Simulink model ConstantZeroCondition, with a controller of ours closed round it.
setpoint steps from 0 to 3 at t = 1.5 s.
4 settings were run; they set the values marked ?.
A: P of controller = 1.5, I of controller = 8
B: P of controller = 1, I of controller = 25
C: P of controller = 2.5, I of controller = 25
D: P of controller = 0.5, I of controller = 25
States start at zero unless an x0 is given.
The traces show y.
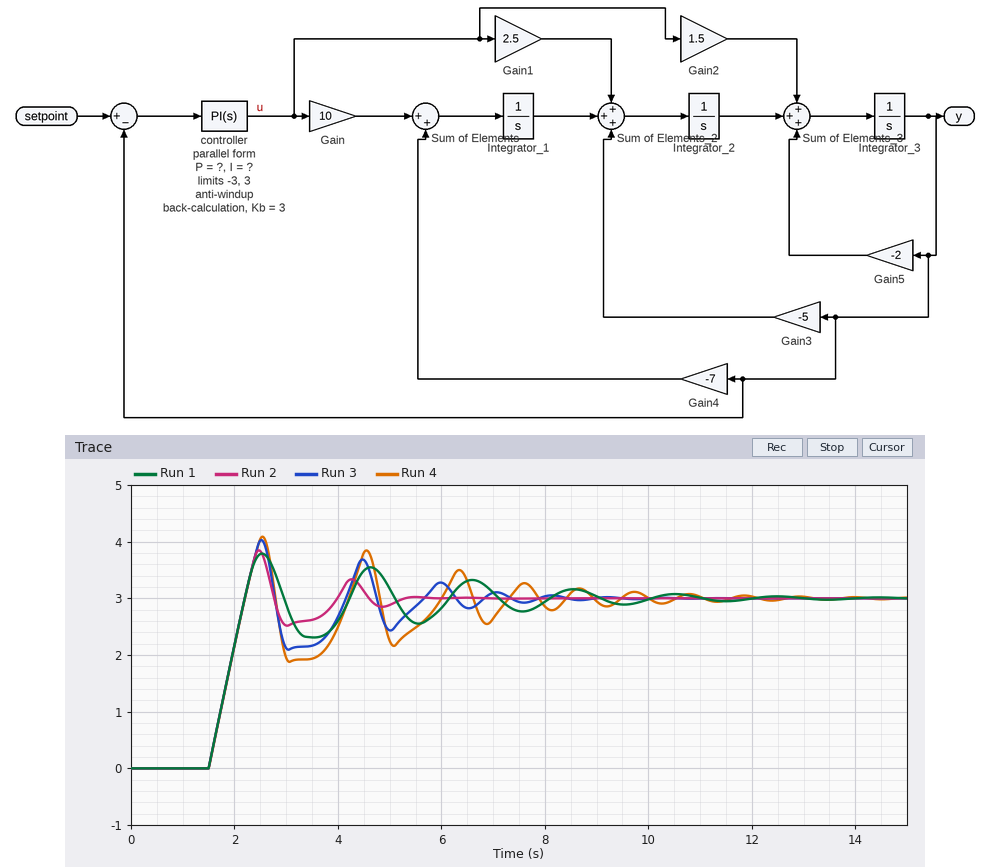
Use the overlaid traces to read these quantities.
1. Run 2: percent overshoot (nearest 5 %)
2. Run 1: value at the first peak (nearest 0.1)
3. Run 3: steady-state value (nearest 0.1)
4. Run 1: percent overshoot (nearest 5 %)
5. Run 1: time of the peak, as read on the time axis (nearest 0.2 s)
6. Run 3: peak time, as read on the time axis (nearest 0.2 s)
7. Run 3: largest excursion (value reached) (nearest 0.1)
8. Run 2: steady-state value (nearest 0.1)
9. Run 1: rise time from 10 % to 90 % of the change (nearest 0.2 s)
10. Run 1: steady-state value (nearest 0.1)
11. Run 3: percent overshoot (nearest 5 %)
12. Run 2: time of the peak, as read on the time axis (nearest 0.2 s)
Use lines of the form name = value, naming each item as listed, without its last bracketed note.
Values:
Run 2: percent overshoot = 30 %
Run 1: value at the first peak = 3.8
Run 3: steady-state value = 3.0
Run 1: percent overshoot = 25 %
Run 1: time of the peak, as read on the time axis = 2.6 s
Run 3: peak time, as read on the time axis = 2.6 s
Run 3: largest excursion (value reached) = 4.0
Run 2: steady-state value = 3.0
Run 1: rise time from 10 % to 90 % of the change = 0.6 s
Run 1: steady-state value = 3.0
Run 3: percent overshoot = 35 %
Run 2: time of the peak, as read on the time axis = 2.4 s
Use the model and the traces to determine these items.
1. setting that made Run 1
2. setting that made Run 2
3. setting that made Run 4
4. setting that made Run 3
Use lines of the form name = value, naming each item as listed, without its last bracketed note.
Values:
setting that made Run 1 = A
setting that made Run 2 = C
setting that made Run 4 = D
setting that made Run 3 = B
